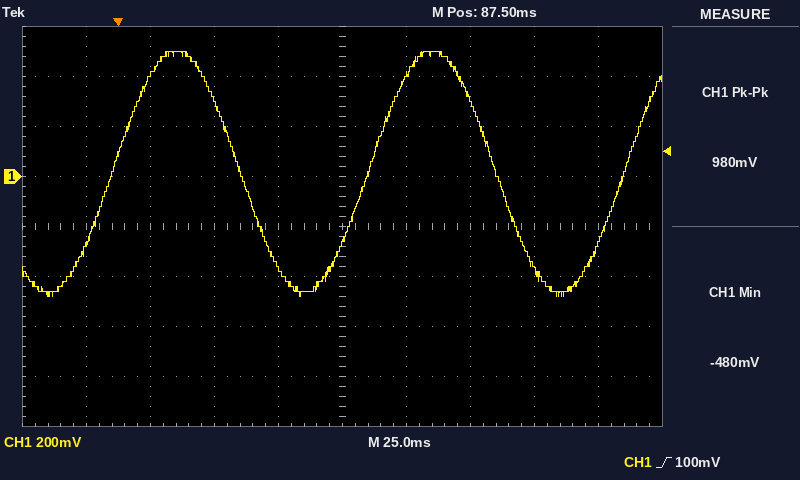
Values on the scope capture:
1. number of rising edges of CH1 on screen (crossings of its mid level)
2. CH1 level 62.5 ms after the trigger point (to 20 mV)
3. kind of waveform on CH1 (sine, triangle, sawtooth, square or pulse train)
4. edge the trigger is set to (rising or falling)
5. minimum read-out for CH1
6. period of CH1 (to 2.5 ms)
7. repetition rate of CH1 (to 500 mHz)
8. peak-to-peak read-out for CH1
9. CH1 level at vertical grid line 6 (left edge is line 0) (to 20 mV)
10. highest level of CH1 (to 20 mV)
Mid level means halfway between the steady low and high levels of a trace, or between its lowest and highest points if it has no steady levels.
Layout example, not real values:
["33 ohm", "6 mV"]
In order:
["3", "-360 mV", "sine", "rising", "-480 mV", "100.0 ms", "10.0 Hz", "980 mV", "400 mV", "500 mV"]
